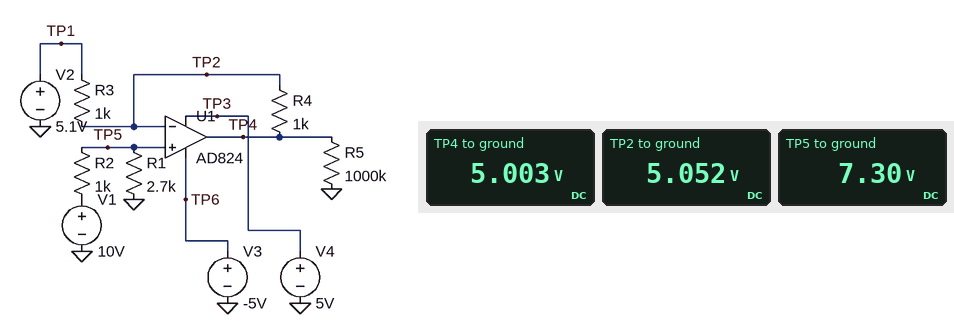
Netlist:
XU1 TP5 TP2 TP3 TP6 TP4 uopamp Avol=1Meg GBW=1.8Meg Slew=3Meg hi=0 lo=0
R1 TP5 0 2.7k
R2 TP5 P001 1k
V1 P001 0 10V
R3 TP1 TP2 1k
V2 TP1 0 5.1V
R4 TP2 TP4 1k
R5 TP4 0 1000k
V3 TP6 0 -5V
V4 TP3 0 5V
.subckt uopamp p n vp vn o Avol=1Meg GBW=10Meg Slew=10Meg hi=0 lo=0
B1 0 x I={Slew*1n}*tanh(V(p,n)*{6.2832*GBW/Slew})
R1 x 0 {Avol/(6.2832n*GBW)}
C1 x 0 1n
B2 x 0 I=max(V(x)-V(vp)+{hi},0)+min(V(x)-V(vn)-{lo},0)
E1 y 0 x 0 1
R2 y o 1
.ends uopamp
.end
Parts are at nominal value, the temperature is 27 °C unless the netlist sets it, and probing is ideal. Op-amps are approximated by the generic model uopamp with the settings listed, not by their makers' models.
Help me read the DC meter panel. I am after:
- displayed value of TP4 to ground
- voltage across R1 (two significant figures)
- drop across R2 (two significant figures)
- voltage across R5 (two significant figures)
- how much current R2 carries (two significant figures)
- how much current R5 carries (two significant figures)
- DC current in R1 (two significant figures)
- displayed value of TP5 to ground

5.003 V
7.3 V
2.7 V
5.0 V
2.7 mA
5.0 µA
2.7 mA
7.30 V
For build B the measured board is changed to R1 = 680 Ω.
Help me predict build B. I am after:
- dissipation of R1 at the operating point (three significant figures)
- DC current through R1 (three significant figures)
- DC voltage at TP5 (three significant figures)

24.1 mW
5.95 mA
4.05 V
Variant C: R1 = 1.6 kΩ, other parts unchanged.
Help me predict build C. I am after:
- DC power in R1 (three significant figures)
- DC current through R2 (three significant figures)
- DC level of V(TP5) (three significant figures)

23.7 mW
3.85 mA
6.15 V
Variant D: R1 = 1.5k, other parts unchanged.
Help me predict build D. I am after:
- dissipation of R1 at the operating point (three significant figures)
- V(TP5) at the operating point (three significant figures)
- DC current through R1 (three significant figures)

24.0 mW
6.00 V
4.00 mA
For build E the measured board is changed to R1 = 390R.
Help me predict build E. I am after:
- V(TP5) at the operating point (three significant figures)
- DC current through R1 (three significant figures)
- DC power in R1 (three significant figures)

2.81 V
7.19 mA
20.2 mW
